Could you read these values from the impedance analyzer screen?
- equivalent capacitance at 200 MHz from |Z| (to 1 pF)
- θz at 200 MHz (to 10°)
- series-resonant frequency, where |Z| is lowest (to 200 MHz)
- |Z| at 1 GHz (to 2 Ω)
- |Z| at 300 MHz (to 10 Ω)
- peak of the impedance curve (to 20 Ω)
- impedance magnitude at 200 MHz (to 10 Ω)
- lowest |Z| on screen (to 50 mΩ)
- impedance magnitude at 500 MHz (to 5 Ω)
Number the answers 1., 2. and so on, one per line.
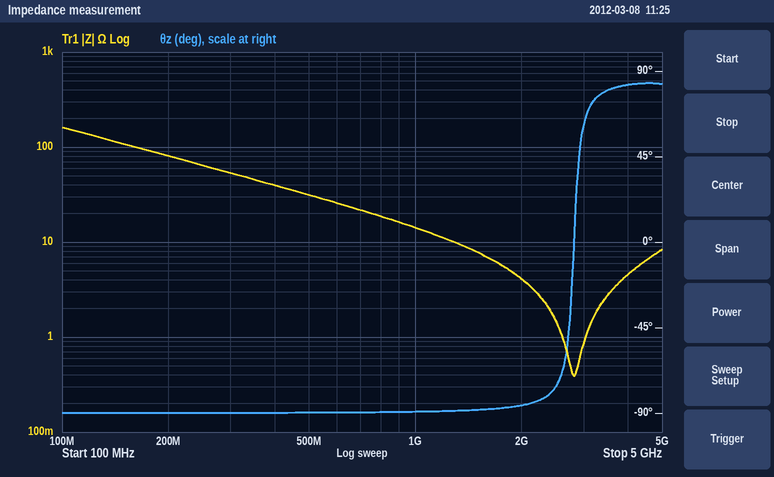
1. 10 pF
2. -90°
3. 2.8 GHz
4. 14 Ω
5. 50 Ω
6. 160 Ω
7. 80 Ω
8. 400 mΩ
9. 30 Ω
